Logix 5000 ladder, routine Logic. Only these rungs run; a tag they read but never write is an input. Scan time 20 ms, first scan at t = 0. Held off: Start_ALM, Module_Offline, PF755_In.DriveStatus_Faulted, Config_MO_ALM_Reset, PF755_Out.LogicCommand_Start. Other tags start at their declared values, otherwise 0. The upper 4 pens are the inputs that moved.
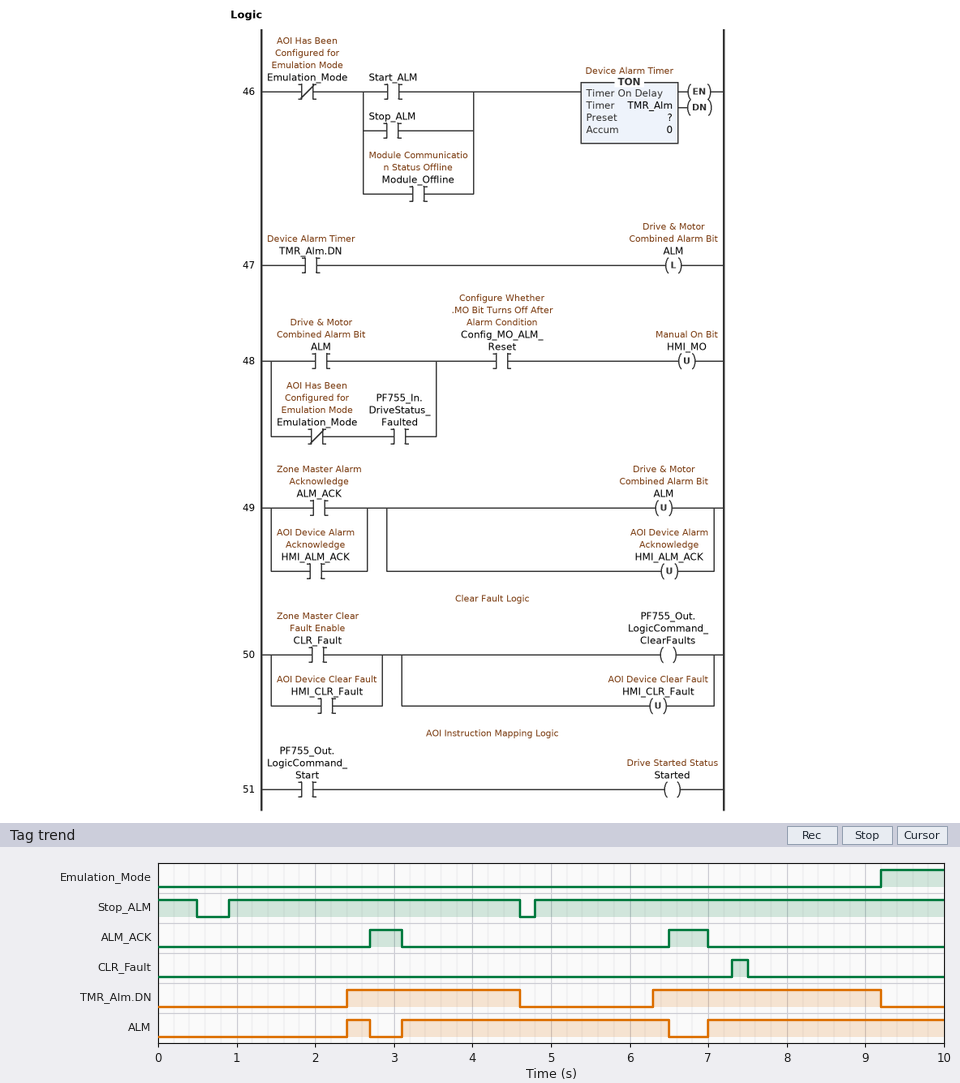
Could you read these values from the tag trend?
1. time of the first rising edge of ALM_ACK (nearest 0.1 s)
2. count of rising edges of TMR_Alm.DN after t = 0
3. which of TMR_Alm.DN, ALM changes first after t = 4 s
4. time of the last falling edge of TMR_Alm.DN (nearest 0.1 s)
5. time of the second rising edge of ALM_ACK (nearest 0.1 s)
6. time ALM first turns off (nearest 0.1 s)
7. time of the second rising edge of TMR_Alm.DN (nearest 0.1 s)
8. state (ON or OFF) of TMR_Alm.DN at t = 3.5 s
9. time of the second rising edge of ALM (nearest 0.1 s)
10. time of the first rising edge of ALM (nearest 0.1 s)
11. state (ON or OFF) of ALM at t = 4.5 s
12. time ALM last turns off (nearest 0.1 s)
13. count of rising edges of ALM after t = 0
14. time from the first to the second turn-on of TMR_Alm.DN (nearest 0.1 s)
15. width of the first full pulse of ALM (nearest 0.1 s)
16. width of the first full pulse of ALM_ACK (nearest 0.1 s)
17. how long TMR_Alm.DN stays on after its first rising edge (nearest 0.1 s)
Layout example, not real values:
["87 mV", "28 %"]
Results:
["2.7 s", "2", "TMR_Alm.DN", "9.2 s", "6.5 s", "2.7 s", "6.3 s", "ON", "3.1 s", "2.4 s", "ON", "6.5 s", "3", "3.9 s", "0.3 s", "0.4 s", "2.2 s"]
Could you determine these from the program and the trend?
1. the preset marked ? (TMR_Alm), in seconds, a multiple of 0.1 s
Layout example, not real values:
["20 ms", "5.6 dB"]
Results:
["1.5 s"]
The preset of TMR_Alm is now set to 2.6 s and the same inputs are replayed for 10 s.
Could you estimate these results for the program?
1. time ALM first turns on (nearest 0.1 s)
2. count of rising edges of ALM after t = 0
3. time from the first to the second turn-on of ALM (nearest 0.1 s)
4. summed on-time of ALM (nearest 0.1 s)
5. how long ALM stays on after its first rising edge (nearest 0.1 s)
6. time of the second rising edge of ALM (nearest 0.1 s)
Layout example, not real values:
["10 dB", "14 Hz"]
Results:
["3.5 s", "2", "3.9 s", "5.6 s", "3.0 s", "7.4 s"]
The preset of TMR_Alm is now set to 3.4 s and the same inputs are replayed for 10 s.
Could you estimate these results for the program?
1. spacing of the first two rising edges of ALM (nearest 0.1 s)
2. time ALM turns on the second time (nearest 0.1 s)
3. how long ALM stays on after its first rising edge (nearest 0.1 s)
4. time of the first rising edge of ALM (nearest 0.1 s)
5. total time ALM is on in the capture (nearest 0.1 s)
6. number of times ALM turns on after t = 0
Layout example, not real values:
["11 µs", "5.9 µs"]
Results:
["3.9 s", "8.2 s", "2.2 s", "4.3 s", "4.0 s", "2"]
